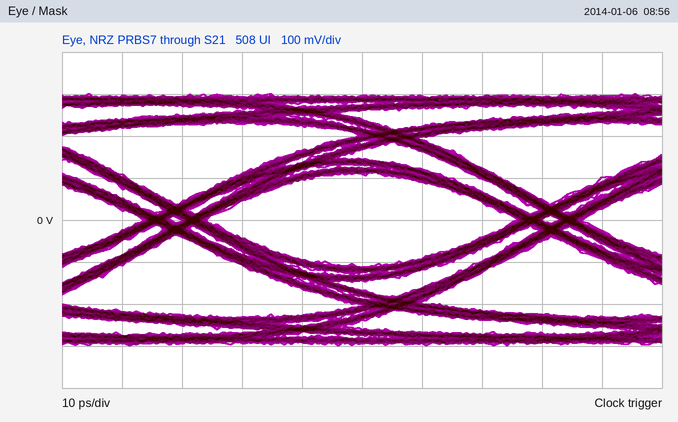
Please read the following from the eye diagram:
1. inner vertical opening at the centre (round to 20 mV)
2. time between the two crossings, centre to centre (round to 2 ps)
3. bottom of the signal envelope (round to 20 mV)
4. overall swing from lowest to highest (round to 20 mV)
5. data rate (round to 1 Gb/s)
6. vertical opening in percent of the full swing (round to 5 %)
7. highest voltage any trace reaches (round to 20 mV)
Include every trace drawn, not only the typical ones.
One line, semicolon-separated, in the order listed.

220 mV; 62 ps; -300 mV; 600 mV; 16 Gb/s; 35 %; 300 mV
